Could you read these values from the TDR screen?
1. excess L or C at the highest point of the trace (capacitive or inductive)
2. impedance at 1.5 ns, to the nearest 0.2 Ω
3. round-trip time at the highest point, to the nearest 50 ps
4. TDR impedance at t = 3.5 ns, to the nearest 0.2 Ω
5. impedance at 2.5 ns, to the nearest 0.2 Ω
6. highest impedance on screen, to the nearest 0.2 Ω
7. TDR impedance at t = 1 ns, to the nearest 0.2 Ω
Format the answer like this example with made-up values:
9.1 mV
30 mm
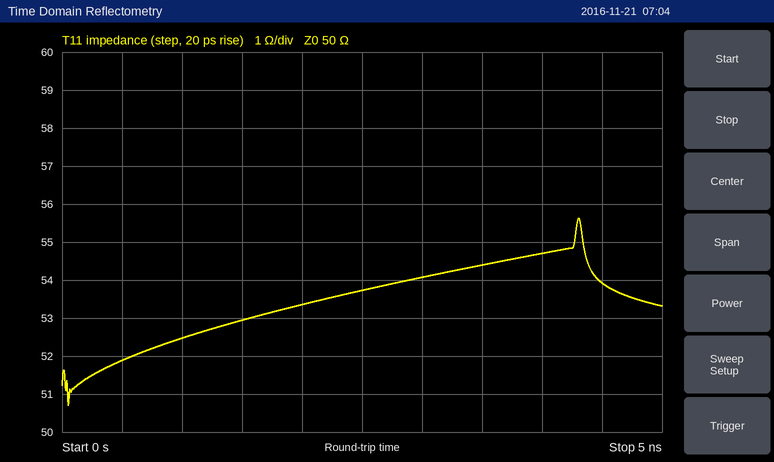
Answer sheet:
inductive
53.0 Ω
4.30 ns
54.4 Ω
53.8 Ω
55.6 Ω
52.4 Ω
